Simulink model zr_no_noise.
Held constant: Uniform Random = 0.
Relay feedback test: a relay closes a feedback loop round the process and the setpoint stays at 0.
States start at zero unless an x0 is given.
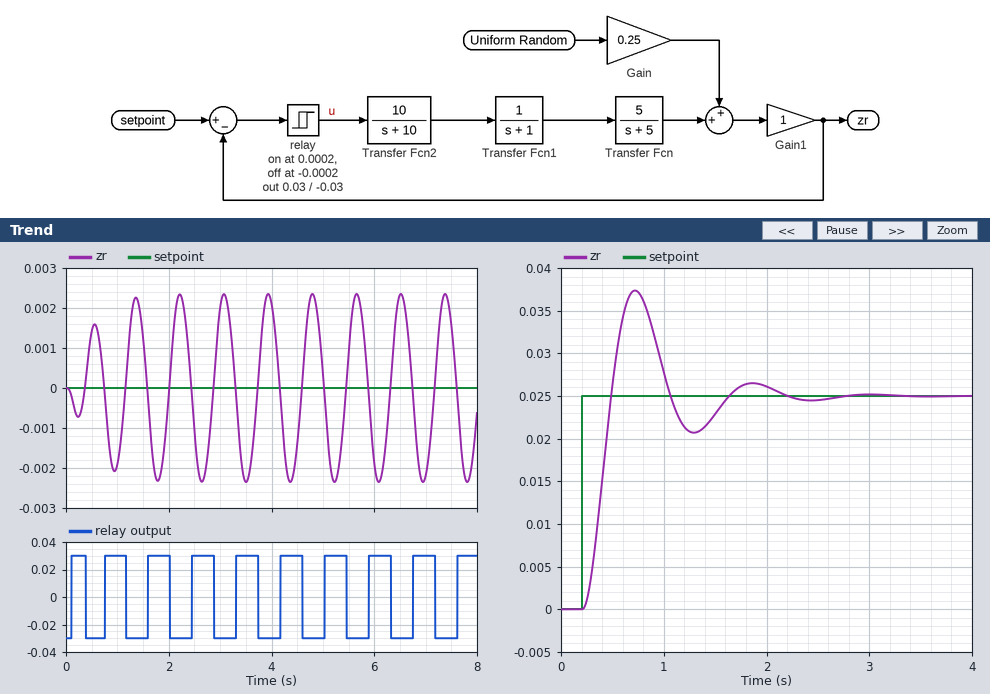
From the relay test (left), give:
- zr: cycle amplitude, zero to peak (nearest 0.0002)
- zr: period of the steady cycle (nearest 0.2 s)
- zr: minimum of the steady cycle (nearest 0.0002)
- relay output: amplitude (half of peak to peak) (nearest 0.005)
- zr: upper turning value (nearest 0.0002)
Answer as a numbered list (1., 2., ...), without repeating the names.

1. 0.0024
2. 0.8 s
3. -0.0024
4. 0.030
5. 0.0024
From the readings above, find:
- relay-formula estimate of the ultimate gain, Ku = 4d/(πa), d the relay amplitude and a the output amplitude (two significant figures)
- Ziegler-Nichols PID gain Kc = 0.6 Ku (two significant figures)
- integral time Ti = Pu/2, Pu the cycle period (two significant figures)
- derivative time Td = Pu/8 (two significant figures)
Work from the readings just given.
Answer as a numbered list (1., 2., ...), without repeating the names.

1. 16
2. 9.6
3. 0.40 s
4. 0.10 s
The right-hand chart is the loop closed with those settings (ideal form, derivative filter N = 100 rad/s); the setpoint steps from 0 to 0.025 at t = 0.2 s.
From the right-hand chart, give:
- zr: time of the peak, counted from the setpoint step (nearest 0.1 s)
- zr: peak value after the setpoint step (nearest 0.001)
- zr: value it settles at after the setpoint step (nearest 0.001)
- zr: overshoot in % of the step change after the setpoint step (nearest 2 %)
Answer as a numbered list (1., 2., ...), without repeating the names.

1. 0.5 s
2. 0.037
3. 0.025
4. 50 %
